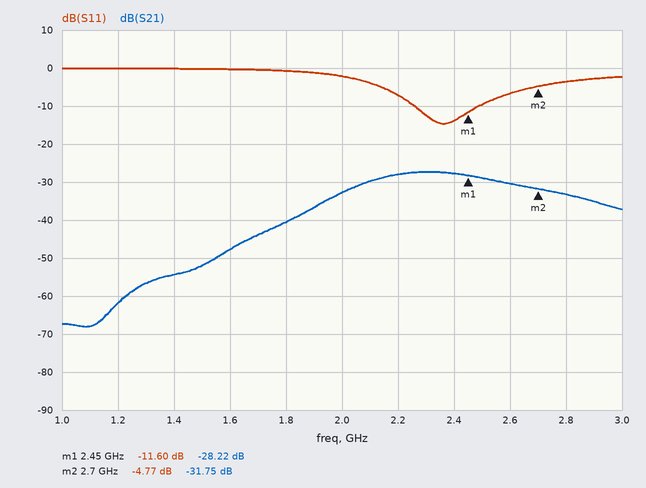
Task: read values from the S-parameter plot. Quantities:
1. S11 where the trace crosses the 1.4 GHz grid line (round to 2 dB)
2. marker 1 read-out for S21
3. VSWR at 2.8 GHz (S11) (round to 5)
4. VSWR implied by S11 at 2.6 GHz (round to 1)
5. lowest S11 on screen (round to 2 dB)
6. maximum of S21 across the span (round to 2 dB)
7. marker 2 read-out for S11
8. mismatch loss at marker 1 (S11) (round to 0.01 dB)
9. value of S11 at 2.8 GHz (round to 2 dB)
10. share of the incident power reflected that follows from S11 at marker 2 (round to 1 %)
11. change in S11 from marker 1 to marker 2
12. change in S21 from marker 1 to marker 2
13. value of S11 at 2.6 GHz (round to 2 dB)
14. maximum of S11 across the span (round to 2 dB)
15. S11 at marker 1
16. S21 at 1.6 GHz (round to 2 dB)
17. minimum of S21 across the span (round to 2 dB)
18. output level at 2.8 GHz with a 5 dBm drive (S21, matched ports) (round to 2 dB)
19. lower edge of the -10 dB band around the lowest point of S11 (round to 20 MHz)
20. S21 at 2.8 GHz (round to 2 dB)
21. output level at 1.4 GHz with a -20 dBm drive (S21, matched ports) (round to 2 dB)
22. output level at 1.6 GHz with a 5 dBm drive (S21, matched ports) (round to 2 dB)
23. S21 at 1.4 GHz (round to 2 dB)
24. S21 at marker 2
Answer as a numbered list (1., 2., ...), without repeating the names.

1. 0 dB
2. -28.22 dB
3. 5
4. 3
5. -14 dB
6. -28 dB
7. -4.77 dB
8. 0.31 dB
9. -4 dB
10. 33 %
11. 6.83 dB
12. -3.53 dB
13. -6 dB
14. 0 dB
15. -11.60 dB
16. -48 dB
17. -68 dB
18. -28 dBm
19. 2.26 GHz
20. -34 dB
21. -74 dBm
22. -42 dBm
23. -54 dB
24. -31.75 dB
